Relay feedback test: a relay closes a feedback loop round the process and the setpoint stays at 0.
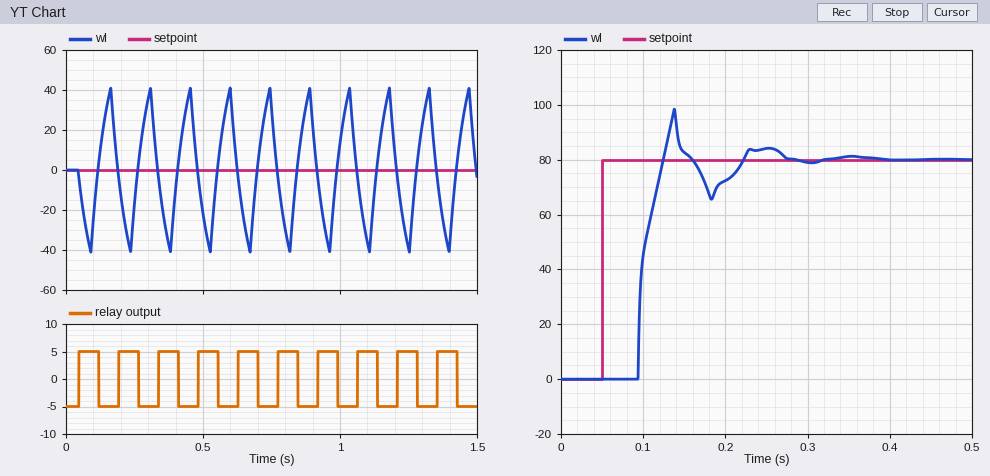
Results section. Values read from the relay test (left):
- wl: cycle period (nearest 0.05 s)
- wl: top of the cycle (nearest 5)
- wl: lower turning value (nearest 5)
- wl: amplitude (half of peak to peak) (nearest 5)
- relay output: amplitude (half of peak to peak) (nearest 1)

0.15 s
40
-40
40
5
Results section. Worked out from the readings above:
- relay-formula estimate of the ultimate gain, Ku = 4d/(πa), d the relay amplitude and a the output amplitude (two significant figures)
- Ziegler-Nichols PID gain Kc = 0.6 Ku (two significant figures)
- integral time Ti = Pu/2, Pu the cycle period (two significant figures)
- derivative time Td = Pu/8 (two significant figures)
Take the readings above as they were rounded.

0.16
0.096
0.075 s
0.019 s
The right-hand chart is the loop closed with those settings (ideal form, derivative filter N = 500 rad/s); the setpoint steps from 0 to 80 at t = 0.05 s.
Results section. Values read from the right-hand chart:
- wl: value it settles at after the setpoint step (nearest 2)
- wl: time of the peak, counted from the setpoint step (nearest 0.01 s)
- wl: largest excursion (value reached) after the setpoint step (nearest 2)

80
0.09 s
98
